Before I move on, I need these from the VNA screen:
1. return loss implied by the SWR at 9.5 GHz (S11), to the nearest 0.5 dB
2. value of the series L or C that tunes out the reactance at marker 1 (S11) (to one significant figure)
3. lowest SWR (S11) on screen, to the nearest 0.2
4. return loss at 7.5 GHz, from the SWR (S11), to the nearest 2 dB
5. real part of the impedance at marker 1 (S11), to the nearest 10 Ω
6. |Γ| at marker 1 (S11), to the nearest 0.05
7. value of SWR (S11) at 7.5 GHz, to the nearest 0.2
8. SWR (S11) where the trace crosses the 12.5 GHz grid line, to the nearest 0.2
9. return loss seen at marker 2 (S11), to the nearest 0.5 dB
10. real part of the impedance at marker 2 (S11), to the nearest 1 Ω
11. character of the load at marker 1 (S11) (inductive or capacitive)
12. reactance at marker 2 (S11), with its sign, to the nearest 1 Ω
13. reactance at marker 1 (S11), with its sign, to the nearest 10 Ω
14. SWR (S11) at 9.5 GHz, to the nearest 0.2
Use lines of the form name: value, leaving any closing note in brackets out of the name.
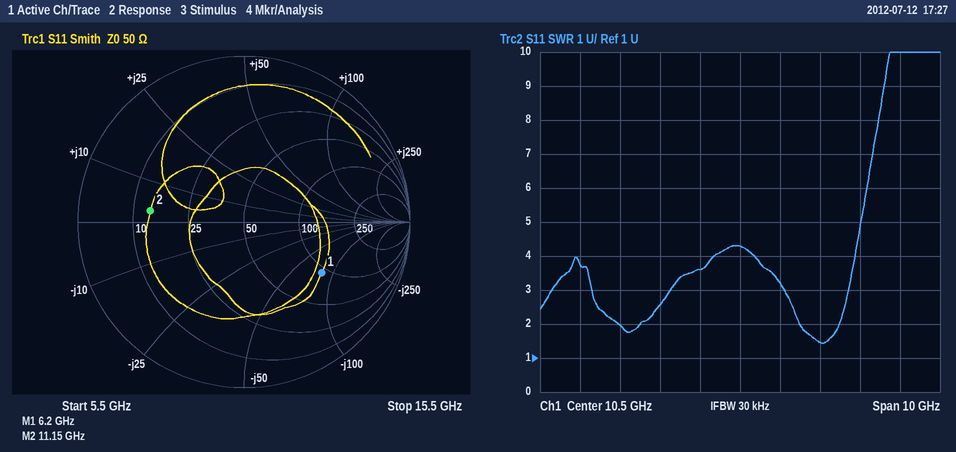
return loss implied by the SWR at 9.5 GHz (S11), to the nearest 0.5 dB: 5.0 dB
value of the series L or C that tunes out the reactance at marker 1 (S11): 2 nH
lowest SWR (S11) on screen, to the nearest 0.2: 1.4
return loss at 7.5 GHz, from the SWR (S11), to the nearest 2 dB: 10 dB
real part of the impedance at marker 1 (S11), to the nearest 10 Ω: 90 Ω
|Γ| at marker 1 (S11), to the nearest 0.05: 0.55
value of SWR (S11) at 7.5 GHz, to the nearest 0.2: 2.0
SWR (S11) where the trace crosses the 12.5 GHz grid line, to the nearest 0.2: 1.4
return loss seen at marker 2 (S11), to the nearest 0.5 dB: 5.0 dB
real part of the impedance at marker 2 (S11), to the nearest 1 Ω: 14 Ω
character of the load at marker 1 (S11): capacitive
reactance at marker 2 (S11), with its sign, to the nearest 1 Ω: +3 Ω
reactance at marker 1 (S11), with its sign, to the nearest 10 Ω: -80 Ω
SWR (S11) at 9.5 GHz, to the nearest 0.2: 3.6
